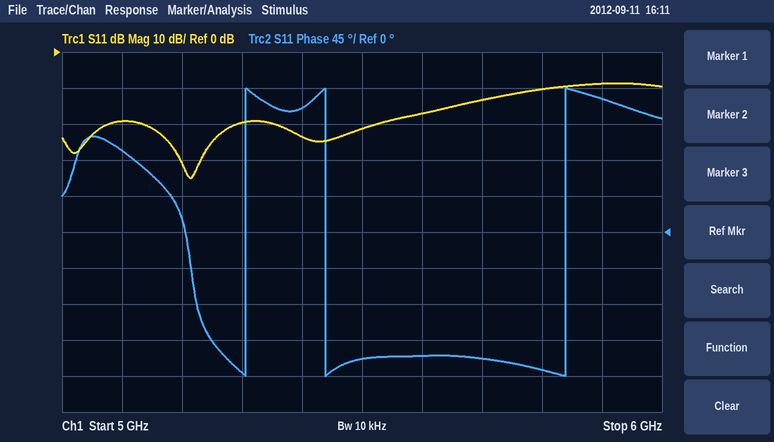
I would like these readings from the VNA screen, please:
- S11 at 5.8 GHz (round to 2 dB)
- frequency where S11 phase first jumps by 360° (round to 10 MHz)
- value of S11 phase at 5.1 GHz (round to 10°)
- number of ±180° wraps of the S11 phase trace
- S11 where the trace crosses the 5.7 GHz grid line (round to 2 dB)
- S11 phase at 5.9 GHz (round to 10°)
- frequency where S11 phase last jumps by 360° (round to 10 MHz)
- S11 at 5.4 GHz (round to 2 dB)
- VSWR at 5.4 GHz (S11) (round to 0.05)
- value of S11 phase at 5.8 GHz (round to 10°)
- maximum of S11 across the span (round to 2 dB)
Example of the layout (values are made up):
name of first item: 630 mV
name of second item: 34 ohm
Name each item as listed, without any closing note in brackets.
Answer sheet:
S11 at 5.8 GHz: -10 dB
frequency where S11 phase first jumps by 360°: 5.31 GHz
value of S11 phase at 5.1 GHz: 100°
number of ±180° wraps of the S11 phase trace: 3
S11 where the trace crosses the 5.7 GHz grid line: -14 dB
S11 phase at 5.9 GHz: 170°
frequency where S11 phase last jumps by 360°: 5.84 GHz
S11 at 5.4 GHz: -24 dB
VSWR at 5.4 GHz (S11): 1.15
value of S11 phase at 5.8 GHz: -170°
maximum of S11 across the span: -8 dB
